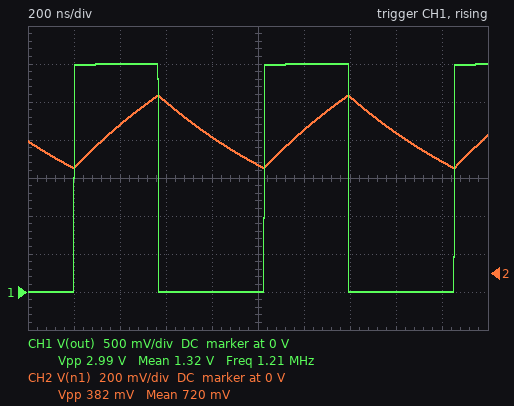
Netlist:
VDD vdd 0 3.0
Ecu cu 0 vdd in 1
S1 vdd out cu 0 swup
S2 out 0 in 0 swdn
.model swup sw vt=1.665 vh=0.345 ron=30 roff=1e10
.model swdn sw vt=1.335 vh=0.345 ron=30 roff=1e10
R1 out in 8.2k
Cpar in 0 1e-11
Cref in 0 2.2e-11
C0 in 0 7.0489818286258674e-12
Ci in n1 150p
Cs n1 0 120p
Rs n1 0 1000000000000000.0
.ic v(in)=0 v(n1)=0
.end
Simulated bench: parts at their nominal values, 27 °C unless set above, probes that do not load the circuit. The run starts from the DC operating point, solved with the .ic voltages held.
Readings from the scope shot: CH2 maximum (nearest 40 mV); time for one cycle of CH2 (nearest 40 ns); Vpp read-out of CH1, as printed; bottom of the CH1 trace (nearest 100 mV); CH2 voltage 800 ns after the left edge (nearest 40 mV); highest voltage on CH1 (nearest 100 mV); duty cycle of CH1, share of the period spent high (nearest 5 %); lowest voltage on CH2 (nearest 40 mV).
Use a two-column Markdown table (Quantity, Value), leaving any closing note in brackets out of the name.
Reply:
| Quantity | Value |
|---|---|
| CH2 maximum | 920 mV |
| time for one cycle of CH2 | 840 ns |
| Vpp read-out of CH1, as printed | 2.99 V |
| bottom of the CH1 trace | 0 V |
| CH2 voltage 800 ns after the left edge | 720 mV |
| highest voltage on CH1 | 3.0 V |
| duty cycle of CH1, share of the period spent high | 45 % |
| lowest voltage on CH2 | 560 mV |
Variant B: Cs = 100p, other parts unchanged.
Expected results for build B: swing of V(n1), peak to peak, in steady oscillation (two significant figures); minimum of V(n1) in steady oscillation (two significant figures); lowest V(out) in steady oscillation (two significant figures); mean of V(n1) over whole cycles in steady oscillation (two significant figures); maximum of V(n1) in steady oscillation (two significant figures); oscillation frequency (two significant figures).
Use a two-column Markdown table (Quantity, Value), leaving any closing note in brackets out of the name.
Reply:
| Quantity | Value |
|---|---|
| swing of V(n1), peak to peak, in steady oscillation | 410 mV |
| minimum of V(n1) in steady oscillation | 590 mV |
| lowest V(out) in steady oscillation | 3.6 mV |
| mean of V(n1) over whole cycles in steady oscillation | 800 mV |
| maximum of V(n1) in steady oscillation | 1.0 V |
| oscillation frequency | 1.3 MHz |
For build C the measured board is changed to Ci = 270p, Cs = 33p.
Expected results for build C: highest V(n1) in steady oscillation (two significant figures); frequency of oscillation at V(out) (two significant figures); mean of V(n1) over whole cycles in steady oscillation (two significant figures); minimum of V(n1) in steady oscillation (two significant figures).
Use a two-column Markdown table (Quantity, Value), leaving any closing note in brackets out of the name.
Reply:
| Quantity | Value |
|---|---|
| highest V(n1) in steady oscillation | 1.5 V |
| frequency of oscillation at V(out) | 1.9 MHz |
| mean of V(n1) over whole cycles in steady oscillation | 1.2 V |
| minimum of V(n1) in steady oscillation | 880 mV |
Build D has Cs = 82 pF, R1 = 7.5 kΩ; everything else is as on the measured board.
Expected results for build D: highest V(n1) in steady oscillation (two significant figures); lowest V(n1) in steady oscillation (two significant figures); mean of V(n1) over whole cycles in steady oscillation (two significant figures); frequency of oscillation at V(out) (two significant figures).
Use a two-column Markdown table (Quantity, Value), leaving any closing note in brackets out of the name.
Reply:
| Quantity | Value |
|---|---|
| highest V(n1) in steady oscillation | 1.1 V |
| lowest V(n1) in steady oscillation | 640 mV |
| mean of V(n1) over whole cycles in steady oscillation | 860 mV |
| frequency of oscillation at V(out) | 1.5 MHz |
